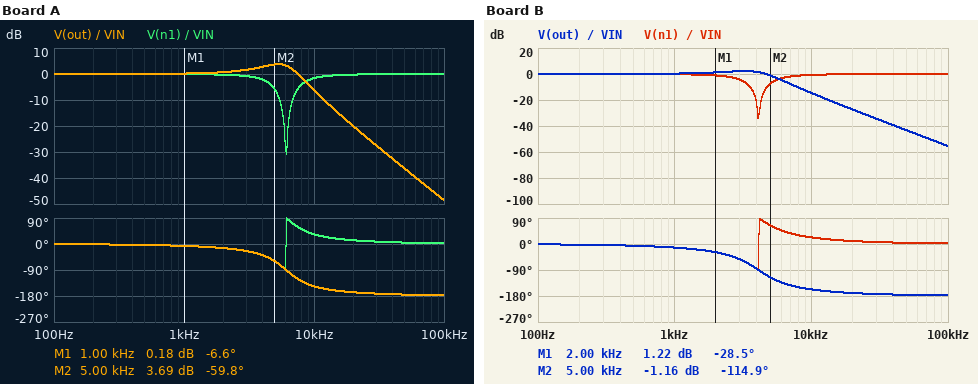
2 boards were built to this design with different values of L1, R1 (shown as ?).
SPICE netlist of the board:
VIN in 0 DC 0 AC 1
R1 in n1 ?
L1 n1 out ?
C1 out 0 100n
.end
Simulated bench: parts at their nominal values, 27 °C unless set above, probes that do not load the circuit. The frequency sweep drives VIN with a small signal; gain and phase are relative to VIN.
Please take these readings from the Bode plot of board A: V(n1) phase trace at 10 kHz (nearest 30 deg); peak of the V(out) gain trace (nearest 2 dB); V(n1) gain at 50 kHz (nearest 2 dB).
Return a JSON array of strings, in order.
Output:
["30 deg", "4 dB", "0 dB"]
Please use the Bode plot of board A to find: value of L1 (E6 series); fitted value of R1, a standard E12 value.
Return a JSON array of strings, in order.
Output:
["6.8 mH", "180 Ω"]
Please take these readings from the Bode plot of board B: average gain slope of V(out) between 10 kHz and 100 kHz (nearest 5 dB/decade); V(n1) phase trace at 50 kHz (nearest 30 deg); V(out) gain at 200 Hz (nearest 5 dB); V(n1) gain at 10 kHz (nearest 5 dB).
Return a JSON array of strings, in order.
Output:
["-40 dB/decade", "0 deg", "0 dB", "0 dB"]
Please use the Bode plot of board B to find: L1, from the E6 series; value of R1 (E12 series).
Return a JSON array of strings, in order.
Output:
["15 mH", "330 Ω"]
